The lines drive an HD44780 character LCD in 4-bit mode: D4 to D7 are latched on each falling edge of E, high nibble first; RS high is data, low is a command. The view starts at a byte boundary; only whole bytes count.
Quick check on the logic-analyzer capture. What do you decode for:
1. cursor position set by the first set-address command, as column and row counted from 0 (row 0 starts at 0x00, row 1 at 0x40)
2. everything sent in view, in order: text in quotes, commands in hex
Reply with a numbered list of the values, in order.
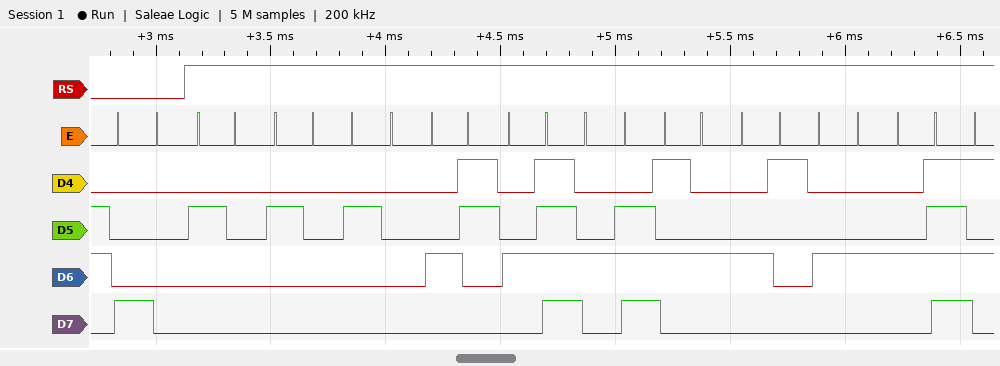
1. column 0, row 0
2. 0x80 "   CONTADO"
